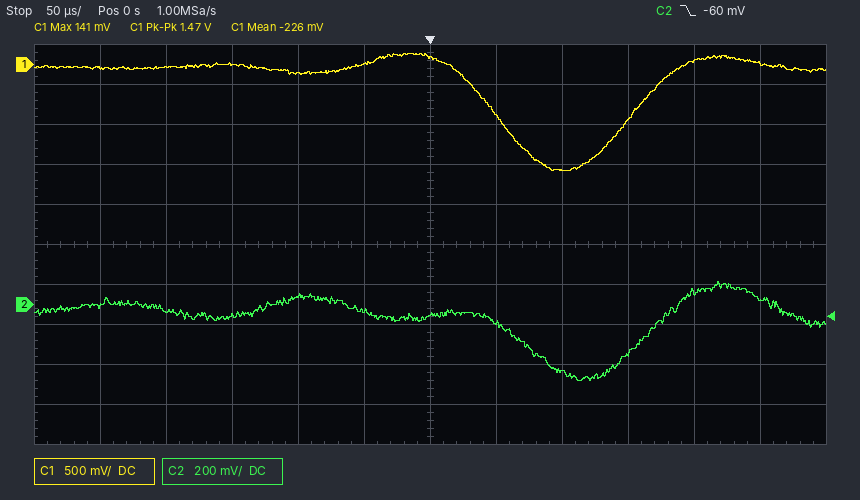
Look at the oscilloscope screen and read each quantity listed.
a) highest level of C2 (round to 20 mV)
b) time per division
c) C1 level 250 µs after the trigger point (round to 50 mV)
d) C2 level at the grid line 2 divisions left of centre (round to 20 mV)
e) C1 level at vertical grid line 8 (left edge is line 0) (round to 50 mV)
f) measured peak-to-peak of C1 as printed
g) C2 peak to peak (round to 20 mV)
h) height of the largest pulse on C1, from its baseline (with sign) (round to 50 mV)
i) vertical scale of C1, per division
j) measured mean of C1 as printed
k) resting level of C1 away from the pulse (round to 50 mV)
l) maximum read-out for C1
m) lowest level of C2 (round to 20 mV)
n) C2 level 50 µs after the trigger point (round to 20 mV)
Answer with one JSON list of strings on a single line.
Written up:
["120 mV", "50 µs", "0 mV", "40 mV", "-1.30 V", "1.47 V", "500 mV", "-1.30 V", "500 mV", "-226 mV", "-50 mV", "141 mV", "-380 mV", "-100 mV"]
